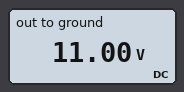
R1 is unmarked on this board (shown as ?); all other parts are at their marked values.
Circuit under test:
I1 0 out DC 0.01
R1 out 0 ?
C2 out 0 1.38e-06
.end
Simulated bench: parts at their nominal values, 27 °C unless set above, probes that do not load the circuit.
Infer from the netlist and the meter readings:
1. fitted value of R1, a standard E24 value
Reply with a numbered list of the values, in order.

1. 1.1 kΩ
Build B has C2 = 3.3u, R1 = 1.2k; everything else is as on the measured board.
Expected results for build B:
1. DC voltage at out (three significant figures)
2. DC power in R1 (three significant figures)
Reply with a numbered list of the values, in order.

1. 12.0 V
2. 120 mW
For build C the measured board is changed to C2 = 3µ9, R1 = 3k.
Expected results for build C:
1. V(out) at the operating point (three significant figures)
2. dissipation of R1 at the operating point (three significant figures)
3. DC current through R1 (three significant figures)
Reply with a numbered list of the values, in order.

1. 30.0 V
2. 300 mW
3. 10.0 mA
